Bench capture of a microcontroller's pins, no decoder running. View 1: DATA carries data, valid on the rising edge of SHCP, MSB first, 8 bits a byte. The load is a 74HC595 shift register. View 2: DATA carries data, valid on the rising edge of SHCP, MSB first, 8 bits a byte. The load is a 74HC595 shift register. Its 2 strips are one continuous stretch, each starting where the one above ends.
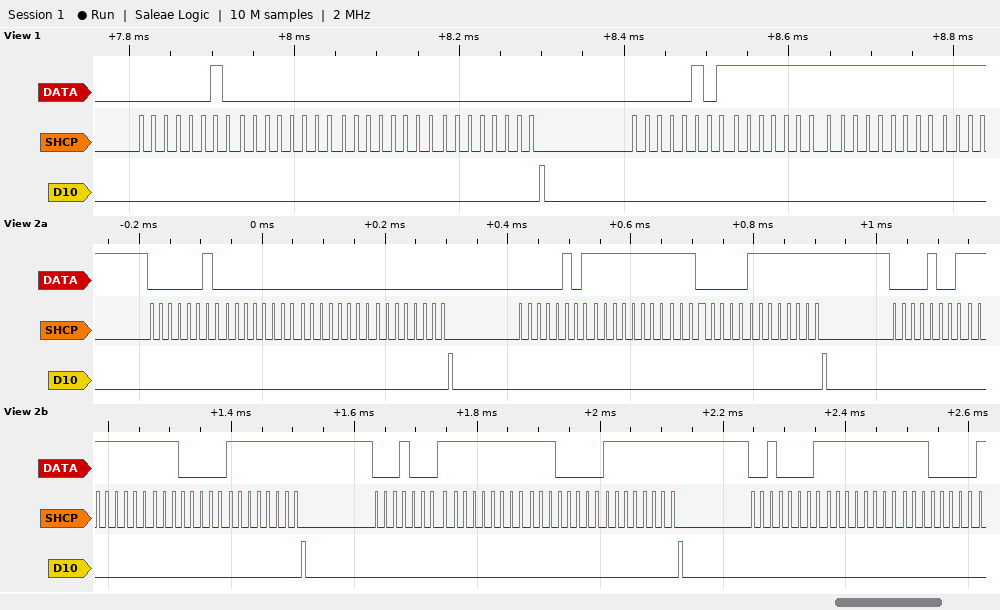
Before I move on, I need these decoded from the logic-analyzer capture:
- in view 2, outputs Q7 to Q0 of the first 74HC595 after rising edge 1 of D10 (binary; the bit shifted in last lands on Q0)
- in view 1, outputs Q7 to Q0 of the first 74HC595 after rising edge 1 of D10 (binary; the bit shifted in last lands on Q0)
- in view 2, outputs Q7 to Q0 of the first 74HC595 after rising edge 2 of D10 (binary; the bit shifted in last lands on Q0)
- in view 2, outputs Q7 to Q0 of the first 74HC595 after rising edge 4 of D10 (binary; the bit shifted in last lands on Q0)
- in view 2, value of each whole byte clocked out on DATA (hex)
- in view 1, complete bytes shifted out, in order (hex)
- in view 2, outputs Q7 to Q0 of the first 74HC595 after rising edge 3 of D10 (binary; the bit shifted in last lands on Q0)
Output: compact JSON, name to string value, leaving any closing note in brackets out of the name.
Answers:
{"in view 2, outputs Q7 to Q0 of the first 74HC595 after rising edge 1 of D10": "00000000", "in view 1, outputs Q7 to Q0 of the first 74HC595 after rising edge 1 of D10": "00000000", "in view 2, outputs Q7 to Q0 of the first 74HC595 after rising edge 2 of D10": "11111111", "in view 2, outputs Q7 to Q0 of the first 74HC595 after rising edge 4 of D10": "11111111", "in view 2, value of each whole byte clocked out on DATA": "02 00 00 00 05 FF E0 FF 09 FF E0 FF 11 FF E0 FF 21 FF E0", "in view 1, complete bytes shifted out, in order": "02 00 00 00 05 FF FF", "in view 2, outputs Q7 to Q0 of the first 74HC595 after rising edge 3 of D10": "11111111"}
